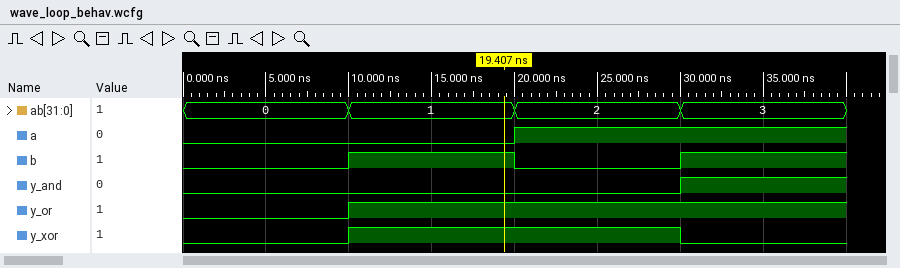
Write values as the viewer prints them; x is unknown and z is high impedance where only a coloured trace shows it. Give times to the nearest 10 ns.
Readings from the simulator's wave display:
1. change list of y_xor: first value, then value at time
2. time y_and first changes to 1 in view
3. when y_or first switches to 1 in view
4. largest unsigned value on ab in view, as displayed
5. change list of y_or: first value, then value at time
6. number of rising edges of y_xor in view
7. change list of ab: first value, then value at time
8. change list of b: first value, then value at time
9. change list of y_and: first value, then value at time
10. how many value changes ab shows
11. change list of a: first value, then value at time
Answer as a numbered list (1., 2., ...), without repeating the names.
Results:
1. 0, 1 at 10 ns, 0 at 30 ns
2. 30 ns
3. 10 ns
4. 3
5. 0, 1 at 10 ns
6. 1
7. 0, 1 at 10 ns, 2 at 20 ns, 3 at 30 ns
8. 0, 1 at 10 ns, 0 at 20 ns, 1 at 30 ns
9. 0, 1 at 30 ns
10. 3
11. 0, 1 at 20 ns
